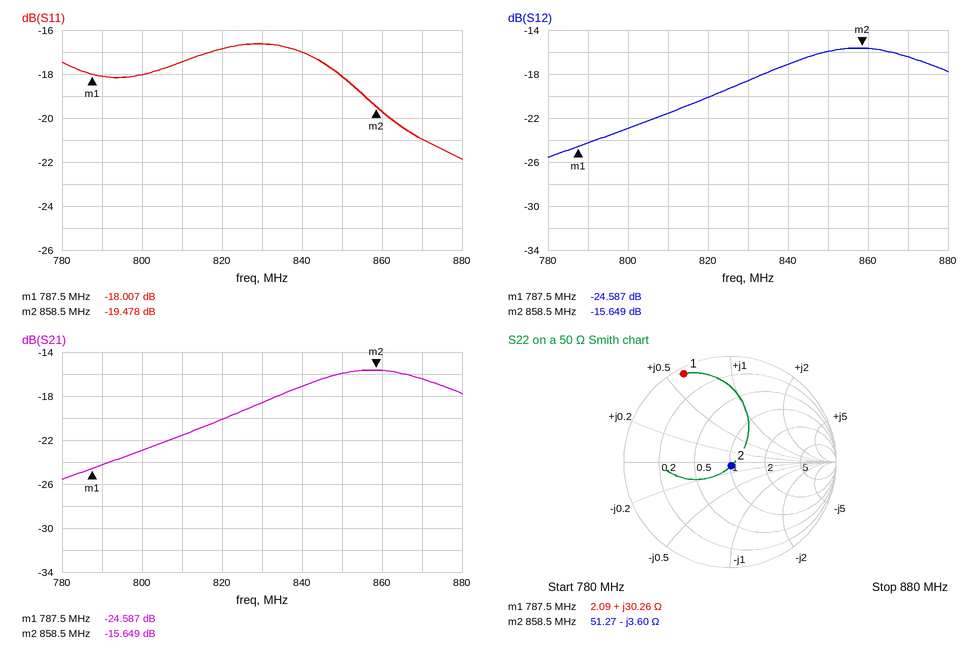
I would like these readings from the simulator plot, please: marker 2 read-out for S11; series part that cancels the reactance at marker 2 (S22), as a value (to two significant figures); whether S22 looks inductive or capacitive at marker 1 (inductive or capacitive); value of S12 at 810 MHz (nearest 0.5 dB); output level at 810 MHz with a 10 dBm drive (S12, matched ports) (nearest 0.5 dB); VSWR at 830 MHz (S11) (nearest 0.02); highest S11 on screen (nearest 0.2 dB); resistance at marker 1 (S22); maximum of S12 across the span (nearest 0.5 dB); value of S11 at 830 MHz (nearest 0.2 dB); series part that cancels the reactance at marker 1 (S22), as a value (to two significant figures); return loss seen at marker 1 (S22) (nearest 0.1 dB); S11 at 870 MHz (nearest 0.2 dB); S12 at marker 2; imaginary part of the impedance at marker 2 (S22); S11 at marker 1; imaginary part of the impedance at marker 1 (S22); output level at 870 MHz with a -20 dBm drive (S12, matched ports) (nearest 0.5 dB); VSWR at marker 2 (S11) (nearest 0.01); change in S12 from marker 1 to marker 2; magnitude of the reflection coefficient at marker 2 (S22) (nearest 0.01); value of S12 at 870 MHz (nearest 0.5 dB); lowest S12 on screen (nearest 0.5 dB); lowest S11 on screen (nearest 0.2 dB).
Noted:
-19.478 dB
670 pH
inductive
-21.5 dB
-11.5 dBm
1.34
-16.6 dB
2.09 Ω
-15.5 dB
-16.6 dB
6.7 pF
0.5 dB
-21.0 dB
-15.649 dB
-3.60 Ω
-18.007 dB
+30.26 Ω
-36.5 dBm
1.24
8.938 dB
0.04
-16.5 dB
-25.5 dB
-21.8 dB
